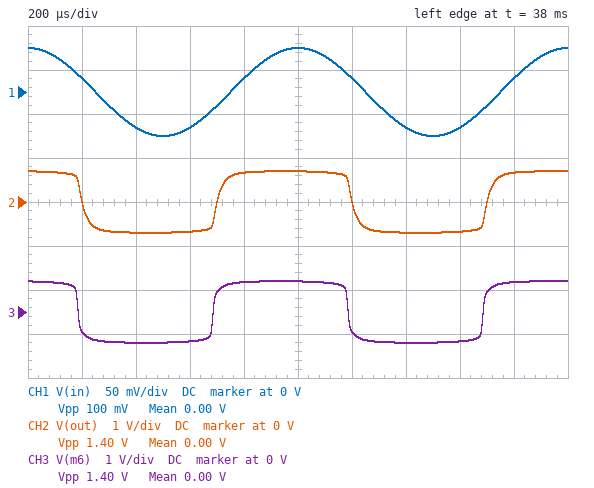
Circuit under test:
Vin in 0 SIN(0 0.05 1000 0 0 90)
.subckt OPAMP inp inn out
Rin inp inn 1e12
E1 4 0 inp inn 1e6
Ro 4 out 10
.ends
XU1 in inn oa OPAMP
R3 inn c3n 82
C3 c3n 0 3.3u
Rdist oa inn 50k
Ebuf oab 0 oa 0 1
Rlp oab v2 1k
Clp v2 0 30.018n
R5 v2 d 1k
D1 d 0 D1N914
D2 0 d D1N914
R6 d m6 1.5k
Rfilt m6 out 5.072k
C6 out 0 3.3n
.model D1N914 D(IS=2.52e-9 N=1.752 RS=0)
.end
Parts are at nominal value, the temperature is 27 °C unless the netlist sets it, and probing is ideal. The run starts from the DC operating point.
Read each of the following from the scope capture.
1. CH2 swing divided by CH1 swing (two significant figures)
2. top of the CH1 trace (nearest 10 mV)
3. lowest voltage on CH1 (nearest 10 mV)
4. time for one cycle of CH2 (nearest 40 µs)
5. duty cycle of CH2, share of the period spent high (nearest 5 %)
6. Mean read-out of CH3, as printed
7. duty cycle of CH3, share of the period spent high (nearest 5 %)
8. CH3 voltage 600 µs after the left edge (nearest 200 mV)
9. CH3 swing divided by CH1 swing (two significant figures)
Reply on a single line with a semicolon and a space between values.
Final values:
14; 50 mV; -50 mV; 1.00 ms; 50 %; 0.00 V; 50 %; -600 mV; 14
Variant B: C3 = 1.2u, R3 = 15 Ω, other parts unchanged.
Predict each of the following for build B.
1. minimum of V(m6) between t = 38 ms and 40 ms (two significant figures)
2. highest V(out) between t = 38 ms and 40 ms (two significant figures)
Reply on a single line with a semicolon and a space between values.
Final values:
-680 mV; 680 mV
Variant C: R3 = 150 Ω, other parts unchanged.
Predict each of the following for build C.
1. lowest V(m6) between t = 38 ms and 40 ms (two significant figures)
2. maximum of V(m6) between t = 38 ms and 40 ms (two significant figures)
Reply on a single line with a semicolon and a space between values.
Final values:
-680 mV; 680 mV
